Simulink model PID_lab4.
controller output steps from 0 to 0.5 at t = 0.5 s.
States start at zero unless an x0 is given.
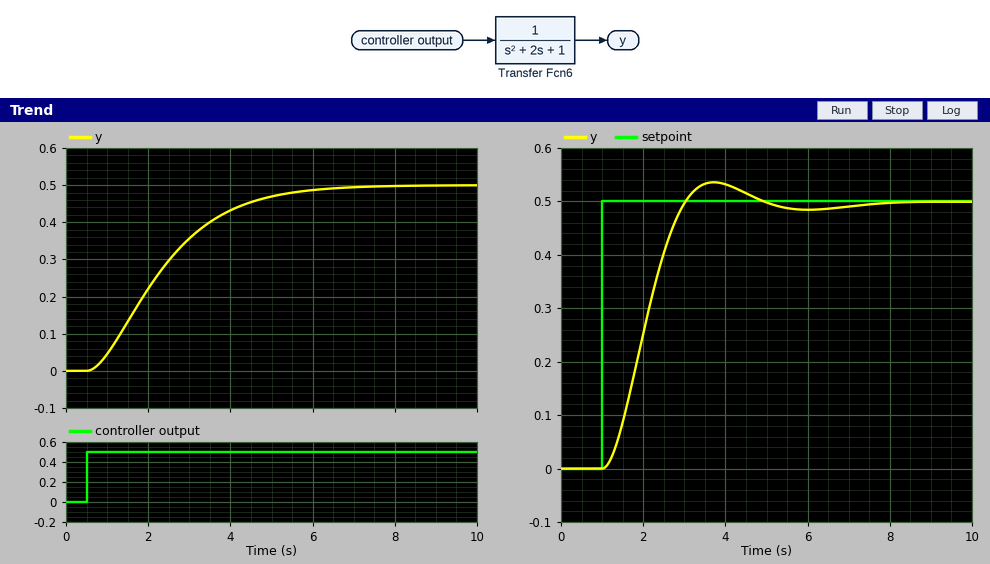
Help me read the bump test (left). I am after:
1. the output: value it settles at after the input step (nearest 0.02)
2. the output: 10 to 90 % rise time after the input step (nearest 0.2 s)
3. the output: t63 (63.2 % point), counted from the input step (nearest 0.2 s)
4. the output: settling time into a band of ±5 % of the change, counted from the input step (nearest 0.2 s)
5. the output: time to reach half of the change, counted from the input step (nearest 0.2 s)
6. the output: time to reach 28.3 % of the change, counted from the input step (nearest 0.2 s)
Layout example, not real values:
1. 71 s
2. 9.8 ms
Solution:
1. 0.50
2. 3.4 s
3. 2.2 s
4. 4.8 s
5. 1.6 s
6. 1.0 s
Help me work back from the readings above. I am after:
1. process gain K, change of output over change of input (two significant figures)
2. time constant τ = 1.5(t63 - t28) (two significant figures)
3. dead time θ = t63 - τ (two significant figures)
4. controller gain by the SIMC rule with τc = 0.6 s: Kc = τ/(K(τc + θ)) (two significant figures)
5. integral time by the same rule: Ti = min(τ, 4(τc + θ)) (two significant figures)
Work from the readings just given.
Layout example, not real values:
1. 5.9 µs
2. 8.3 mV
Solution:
1. 1.0
2. 1.8 s
3. 0.40 s
4. 1.8
5. 1.8 s
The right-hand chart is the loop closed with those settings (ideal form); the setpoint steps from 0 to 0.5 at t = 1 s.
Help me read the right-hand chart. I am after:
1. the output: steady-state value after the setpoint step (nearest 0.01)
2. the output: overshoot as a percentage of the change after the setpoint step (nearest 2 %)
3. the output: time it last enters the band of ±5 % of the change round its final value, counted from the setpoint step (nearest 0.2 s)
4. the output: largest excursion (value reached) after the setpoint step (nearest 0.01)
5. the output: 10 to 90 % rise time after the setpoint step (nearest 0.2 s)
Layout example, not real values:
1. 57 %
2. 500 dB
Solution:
1. 0.50
2. 8 %
3. 3.2 s
4. 0.54
5. 1.4 s
